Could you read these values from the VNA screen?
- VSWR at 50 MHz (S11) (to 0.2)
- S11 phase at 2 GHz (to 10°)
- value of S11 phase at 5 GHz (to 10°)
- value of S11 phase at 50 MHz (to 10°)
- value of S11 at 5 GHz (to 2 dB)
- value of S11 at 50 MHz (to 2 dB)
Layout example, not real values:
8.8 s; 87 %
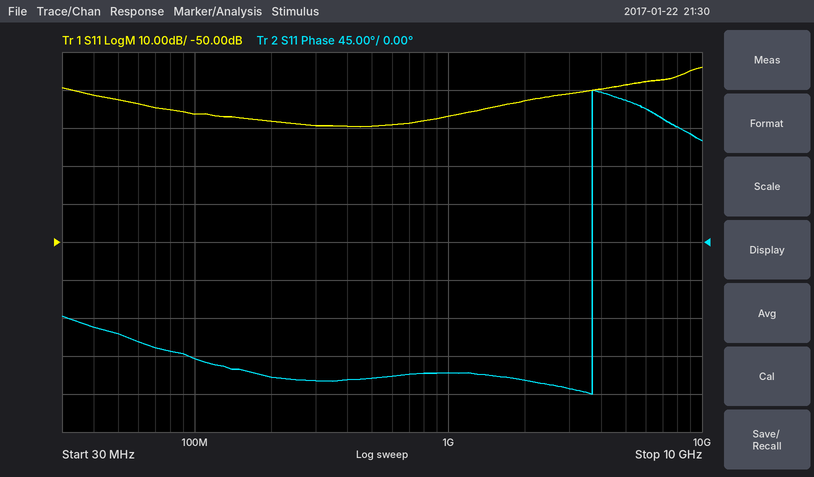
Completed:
1.6; -160°; 170°; -110°; -8 dB; -12 dB
